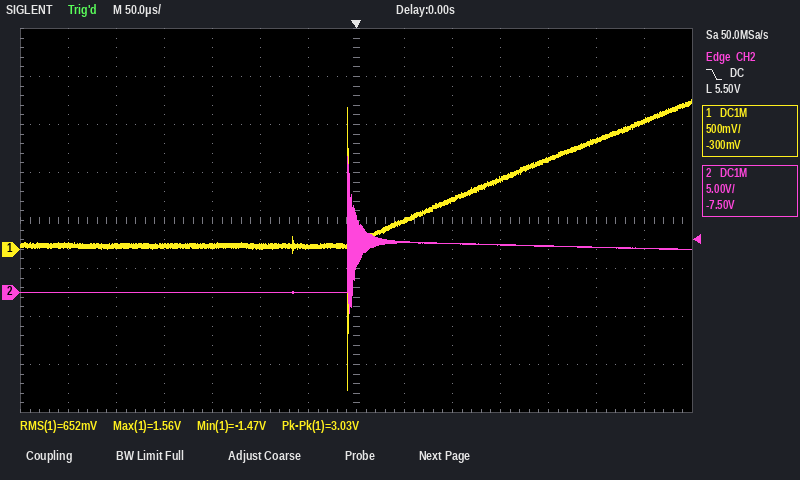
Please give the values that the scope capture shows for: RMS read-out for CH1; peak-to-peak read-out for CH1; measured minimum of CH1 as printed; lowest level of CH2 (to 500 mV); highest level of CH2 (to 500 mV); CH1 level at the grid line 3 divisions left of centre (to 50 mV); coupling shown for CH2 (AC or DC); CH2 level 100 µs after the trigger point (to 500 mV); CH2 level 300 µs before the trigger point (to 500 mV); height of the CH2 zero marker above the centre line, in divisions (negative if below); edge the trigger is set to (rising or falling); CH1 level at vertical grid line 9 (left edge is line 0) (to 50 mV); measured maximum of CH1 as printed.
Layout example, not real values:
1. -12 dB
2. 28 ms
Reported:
1. 652 mV
2. 3.03 V
3. -1.47 V
4. -2.0 V
5. 14.0 V
6. 50 mV
7. DC
8. 5.0 V
9. 0.0 V
10. -1.5 div
11. falling
12. 500 mV
13. 1.56 V
